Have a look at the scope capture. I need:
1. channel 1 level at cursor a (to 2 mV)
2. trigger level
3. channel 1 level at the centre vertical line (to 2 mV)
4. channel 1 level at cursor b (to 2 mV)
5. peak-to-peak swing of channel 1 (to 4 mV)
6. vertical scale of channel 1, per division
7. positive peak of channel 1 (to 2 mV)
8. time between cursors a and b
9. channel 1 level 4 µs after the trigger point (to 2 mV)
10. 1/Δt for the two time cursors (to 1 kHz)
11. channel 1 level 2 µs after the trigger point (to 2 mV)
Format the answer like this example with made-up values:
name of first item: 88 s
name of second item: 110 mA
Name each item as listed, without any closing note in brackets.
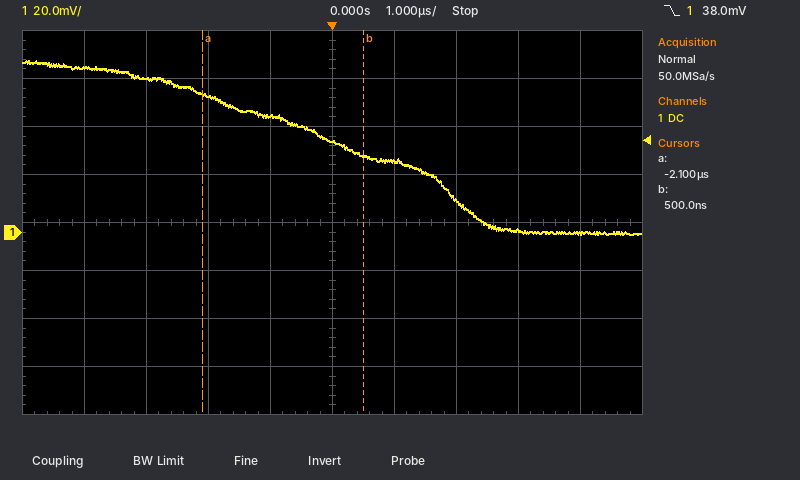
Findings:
channel 1 level at cursor a: 58 mV
trigger level: 38.0 mV
channel 1 level at the centre vertical line: 38 mV
channel 1 level at cursor b: 32 mV
peak-to-peak swing of channel 1: 72 mV
vertical scale of channel 1, per division: 20 mV
positive peak of channel 1: 72 mV
time between cursors a and b: 2.6 µs
channel 1 level 4 µs after the trigger point: 0 mV
1/Δt for the two time cursors: 385 kHz
channel 1 level 2 µs after the trigger point: 14 mV
